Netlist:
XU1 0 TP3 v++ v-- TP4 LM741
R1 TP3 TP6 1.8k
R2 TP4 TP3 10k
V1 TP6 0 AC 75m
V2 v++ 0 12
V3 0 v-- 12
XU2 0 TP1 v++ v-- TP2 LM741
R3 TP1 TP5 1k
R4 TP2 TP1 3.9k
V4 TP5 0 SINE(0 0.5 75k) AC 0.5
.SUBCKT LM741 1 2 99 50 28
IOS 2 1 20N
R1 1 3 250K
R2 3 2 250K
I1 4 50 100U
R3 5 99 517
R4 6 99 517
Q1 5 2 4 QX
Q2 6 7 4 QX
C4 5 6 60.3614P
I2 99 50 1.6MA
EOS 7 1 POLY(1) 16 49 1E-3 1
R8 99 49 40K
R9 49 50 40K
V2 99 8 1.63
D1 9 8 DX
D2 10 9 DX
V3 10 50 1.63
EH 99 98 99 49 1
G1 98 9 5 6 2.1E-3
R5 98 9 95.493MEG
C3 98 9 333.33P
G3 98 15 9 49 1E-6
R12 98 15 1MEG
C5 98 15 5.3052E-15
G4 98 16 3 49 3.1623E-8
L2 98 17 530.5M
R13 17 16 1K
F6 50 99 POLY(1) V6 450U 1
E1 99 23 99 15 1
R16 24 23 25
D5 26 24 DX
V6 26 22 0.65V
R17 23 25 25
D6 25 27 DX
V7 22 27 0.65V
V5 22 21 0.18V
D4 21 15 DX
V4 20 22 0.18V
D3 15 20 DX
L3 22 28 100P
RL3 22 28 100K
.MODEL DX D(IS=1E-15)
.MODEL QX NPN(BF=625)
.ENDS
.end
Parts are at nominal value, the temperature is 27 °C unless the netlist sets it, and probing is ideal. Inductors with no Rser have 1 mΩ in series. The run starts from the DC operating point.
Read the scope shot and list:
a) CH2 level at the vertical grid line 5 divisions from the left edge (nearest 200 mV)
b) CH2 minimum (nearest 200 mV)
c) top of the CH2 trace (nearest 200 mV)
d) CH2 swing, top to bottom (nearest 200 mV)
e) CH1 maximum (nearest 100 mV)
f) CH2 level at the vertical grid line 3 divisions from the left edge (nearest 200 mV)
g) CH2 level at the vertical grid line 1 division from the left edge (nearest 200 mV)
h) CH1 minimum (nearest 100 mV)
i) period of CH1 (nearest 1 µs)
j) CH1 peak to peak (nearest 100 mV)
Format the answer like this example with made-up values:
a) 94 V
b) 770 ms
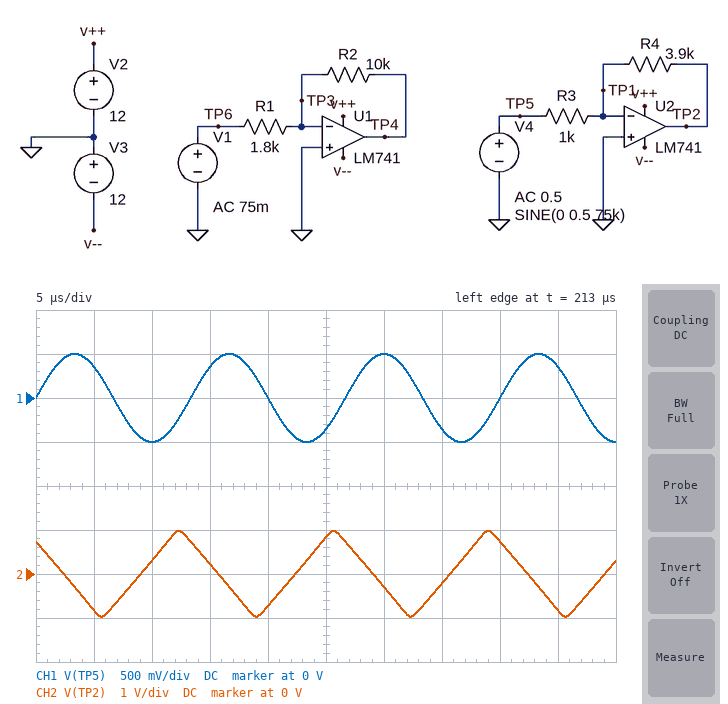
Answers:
a) 800 mV
b) -1.0 V
c) 1.0 V
d) 2.0 V
e) 500 mV
f) 200 mV
g) -800 mV
h) -500 mV
i) 13 µs
j) 1.0 V
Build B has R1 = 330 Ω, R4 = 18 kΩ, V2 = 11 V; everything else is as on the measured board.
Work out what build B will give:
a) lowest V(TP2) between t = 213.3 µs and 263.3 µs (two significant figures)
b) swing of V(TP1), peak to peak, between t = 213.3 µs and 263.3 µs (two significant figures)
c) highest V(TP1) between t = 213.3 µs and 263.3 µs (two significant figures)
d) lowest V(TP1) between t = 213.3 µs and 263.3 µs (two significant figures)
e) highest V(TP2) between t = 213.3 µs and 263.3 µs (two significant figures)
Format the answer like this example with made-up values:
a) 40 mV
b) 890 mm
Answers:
a) -1.0 V
b) 940 mV
c) 470 mV
d) -470 mV
e) 1.0 V
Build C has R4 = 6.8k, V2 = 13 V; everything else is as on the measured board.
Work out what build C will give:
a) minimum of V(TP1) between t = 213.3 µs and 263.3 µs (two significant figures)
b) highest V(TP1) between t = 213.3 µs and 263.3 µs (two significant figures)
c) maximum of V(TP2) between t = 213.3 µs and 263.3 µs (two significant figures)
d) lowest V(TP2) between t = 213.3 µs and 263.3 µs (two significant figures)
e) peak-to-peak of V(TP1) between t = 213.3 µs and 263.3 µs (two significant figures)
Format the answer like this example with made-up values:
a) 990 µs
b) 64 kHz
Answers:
a) -420 mV
b) 420 mV
c) 1.0 V
d) -990 mV
e) 850 mV
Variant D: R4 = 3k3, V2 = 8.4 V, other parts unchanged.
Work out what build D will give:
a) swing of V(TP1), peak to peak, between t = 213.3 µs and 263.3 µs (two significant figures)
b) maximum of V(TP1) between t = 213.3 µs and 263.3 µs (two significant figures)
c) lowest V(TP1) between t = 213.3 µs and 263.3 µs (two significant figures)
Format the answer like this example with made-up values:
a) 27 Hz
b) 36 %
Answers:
a) 660 mV
b) 330 mV
c) -330 mV
